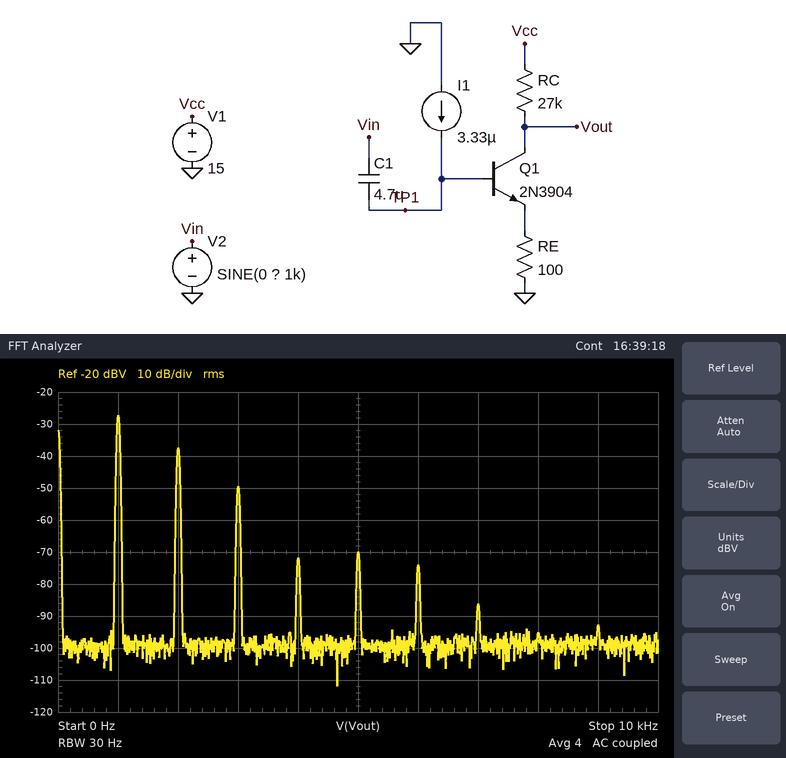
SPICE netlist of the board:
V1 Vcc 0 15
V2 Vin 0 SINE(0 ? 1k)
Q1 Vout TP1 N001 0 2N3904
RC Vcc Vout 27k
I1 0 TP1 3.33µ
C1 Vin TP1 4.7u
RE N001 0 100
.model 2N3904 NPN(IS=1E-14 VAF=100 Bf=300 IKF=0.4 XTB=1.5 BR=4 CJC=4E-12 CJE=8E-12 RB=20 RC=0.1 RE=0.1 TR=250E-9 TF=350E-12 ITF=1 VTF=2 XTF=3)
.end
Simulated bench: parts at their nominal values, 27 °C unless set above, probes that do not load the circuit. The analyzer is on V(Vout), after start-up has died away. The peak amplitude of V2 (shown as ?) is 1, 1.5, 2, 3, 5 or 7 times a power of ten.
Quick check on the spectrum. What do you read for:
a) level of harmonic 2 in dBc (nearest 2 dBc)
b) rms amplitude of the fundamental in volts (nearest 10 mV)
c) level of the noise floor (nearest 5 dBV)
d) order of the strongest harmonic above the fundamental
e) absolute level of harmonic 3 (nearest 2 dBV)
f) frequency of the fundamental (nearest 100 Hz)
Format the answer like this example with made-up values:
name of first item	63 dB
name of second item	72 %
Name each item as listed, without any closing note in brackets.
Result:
level of harmonic 2 in dBc	-10 dBc
rms amplitude of the fundamental in volts	40 mV
level of the noise floor	-100 dBV
order of the strongest harmonic above the fundamental	2
absolute level of harmonic 3	-50 dBV
frequency of the fundamental	1.0 kHz
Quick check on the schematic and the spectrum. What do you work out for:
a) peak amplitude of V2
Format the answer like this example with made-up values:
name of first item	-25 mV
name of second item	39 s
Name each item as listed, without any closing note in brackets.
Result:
peak amplitude of V2	1 mV
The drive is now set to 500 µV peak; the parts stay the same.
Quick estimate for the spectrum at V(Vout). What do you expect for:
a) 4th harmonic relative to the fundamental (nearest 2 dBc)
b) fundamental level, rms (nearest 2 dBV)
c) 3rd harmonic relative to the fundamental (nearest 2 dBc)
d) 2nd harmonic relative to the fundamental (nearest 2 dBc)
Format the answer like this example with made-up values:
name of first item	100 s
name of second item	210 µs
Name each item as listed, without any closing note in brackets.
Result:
4th harmonic relative to the fundamental	-48 dBc
fundamental level, rms	-36 dBV
3rd harmonic relative to the fundamental	-32 dBc
2nd harmonic relative to the fundamental	-16 dBc
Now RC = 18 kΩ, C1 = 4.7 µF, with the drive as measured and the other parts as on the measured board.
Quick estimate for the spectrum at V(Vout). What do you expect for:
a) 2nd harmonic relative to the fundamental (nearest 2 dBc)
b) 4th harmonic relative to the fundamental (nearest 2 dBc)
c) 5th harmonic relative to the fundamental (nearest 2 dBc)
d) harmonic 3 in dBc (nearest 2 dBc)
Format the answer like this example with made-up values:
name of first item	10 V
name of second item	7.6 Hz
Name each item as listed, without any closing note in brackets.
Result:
2nd harmonic relative to the fundamental	-16 dBc
4th harmonic relative to the fundamental	-40 dBc
5th harmonic relative to the fundamental	-48 dBc
harmonic 3 in dBc	-32 dBc
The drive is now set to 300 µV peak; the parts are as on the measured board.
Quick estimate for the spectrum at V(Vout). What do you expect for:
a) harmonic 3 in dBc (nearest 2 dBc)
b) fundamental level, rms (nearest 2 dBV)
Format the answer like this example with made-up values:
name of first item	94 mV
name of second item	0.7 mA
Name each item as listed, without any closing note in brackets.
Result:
harmonic 3 in dBc	-40 dBc
fundamental level, rms	-42 dBV
